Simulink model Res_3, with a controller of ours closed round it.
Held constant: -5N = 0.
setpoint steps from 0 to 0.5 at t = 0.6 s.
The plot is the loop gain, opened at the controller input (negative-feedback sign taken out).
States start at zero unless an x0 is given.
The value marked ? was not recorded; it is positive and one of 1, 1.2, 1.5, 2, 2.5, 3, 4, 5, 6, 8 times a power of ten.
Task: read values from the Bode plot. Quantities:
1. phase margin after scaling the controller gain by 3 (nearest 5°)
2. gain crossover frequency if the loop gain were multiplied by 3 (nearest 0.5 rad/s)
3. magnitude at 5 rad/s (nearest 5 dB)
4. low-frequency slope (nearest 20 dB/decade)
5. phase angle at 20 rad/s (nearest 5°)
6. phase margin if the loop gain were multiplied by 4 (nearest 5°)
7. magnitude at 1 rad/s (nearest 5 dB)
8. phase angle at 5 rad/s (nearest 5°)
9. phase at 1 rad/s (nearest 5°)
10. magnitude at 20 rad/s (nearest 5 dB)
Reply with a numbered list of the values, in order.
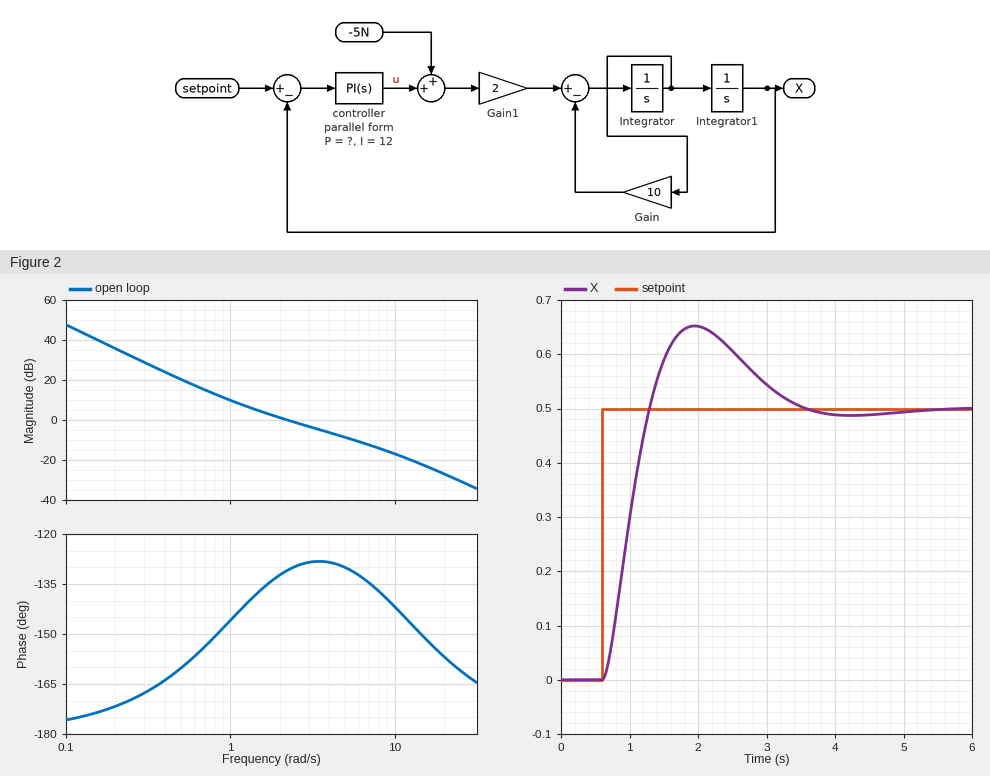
1. 50°
2. 5.5 rad/s
3. -10 dB
4. -40 dB/decade
5. -155°
6. 45°
7. 10 dB
8. -130°
9. -145°
10. -25 dB
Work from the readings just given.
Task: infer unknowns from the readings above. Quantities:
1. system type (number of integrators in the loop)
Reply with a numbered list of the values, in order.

1. 2
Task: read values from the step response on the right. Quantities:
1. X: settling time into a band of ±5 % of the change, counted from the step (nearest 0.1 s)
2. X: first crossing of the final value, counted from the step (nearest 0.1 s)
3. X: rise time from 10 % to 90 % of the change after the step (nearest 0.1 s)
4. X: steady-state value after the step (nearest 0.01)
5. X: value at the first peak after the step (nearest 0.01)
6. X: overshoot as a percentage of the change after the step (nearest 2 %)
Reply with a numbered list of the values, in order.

1. 2.6 s
2. 0.7 s
3. 0.5 s
4. 0.50
5. 0.65
6. 30 %
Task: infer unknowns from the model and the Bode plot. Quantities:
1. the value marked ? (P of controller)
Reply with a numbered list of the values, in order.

1. 10
